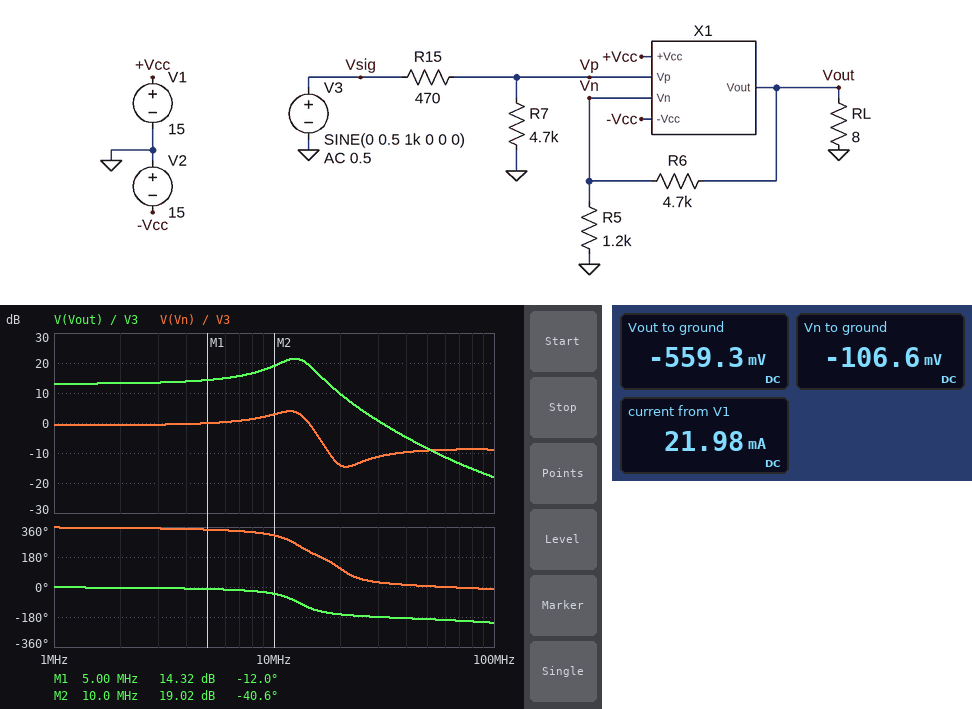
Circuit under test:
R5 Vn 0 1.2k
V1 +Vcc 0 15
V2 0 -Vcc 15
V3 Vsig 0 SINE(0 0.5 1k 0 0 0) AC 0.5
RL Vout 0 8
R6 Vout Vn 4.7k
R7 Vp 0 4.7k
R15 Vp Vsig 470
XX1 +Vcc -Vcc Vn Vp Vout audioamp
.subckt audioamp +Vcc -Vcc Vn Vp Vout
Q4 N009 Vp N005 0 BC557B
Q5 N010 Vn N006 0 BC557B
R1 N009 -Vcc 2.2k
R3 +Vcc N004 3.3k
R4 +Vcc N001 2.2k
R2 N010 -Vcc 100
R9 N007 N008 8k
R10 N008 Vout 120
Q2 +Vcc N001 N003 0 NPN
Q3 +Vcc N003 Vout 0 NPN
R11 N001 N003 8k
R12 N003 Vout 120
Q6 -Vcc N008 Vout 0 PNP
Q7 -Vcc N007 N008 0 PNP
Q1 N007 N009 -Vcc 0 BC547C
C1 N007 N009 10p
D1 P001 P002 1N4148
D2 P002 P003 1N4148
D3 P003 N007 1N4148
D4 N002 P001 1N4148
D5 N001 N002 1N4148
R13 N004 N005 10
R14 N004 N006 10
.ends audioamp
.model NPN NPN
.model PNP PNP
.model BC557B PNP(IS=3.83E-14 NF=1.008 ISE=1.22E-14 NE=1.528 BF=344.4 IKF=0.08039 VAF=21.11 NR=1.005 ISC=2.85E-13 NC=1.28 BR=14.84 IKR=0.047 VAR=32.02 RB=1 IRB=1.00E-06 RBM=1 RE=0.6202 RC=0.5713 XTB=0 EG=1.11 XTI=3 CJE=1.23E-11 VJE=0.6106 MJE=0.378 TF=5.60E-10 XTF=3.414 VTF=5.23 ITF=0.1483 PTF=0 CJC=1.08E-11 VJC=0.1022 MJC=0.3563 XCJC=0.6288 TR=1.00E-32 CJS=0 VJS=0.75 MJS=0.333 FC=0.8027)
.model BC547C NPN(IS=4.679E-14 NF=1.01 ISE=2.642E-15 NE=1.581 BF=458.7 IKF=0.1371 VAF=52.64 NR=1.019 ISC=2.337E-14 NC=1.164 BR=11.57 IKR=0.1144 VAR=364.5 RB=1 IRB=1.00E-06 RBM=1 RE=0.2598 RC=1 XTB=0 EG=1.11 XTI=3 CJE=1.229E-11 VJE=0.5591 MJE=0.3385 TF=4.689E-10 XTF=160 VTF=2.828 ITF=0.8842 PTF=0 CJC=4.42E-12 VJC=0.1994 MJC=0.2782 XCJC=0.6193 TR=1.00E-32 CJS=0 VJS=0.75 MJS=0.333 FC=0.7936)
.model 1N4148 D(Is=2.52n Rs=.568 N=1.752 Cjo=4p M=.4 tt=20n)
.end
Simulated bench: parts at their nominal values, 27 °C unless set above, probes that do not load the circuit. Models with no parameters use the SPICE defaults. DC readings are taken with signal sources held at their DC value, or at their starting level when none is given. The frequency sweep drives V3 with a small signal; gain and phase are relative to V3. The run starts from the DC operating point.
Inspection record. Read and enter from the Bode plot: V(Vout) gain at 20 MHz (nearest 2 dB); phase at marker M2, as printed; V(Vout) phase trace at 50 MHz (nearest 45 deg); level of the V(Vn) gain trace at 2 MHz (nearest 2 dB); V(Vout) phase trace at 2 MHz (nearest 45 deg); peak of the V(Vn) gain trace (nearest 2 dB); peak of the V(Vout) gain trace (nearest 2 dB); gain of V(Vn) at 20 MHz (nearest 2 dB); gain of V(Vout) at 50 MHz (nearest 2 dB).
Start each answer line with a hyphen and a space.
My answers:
- 10 dB
- -40.6 deg
- -180 deg
- 0 dB
- 0 deg
- 4 dB
- 22 dB
- -14 dB
- -8 dB
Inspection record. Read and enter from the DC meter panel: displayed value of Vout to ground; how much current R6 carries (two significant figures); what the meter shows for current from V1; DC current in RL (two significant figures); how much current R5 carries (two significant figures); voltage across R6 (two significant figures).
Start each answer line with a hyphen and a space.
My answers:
- -559.3 mV
- 96 µA
- 21.98 mA
- 70 mA
- 89 µA
- 450 mV
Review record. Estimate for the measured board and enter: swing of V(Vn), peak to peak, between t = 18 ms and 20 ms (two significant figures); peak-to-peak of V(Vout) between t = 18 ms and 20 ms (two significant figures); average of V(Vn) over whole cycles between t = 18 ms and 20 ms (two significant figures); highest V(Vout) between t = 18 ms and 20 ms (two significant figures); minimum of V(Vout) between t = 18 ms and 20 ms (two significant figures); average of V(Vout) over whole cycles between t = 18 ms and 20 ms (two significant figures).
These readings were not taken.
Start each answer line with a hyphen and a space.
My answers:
- 910 mV
- 4.5 V
- -110 mV
- 1.7 V
- -2.8 V
- -560 mV
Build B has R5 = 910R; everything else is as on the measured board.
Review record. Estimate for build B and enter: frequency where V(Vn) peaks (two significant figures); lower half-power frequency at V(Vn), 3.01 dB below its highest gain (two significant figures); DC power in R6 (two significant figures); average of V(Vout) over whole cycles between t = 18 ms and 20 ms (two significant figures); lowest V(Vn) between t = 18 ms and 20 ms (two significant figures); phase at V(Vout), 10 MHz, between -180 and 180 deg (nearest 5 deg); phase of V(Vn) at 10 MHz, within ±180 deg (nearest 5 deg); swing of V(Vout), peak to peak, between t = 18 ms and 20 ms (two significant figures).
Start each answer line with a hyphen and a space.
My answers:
- 11 MHz
- 2.7 MHz
- 73 µW
- -690 mV
- -560 mV
- -55 deg
- -65 deg
- 5.6 V
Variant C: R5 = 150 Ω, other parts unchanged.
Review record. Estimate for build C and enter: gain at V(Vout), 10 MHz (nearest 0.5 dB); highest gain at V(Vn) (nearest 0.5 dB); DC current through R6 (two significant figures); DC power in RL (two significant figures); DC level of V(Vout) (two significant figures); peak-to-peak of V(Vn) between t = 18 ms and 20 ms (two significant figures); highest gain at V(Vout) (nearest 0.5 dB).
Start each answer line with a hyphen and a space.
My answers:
- 20.0 dB
- -1.0 dB
- 710 µA
- 1.5 W
- -3.5 V
- 750 mV
- 29.5 dB
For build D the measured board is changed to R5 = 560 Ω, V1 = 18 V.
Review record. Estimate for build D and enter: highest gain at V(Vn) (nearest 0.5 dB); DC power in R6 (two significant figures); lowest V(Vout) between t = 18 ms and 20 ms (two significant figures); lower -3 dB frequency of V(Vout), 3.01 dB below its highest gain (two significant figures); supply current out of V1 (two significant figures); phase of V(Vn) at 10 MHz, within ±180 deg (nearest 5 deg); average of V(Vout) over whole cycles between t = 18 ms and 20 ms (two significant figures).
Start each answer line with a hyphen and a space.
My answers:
- 0.5 dB
- 240 µW
- -5.5 V
- 630 kHz
- 37 mA
- -90 deg
- -1.2 V
